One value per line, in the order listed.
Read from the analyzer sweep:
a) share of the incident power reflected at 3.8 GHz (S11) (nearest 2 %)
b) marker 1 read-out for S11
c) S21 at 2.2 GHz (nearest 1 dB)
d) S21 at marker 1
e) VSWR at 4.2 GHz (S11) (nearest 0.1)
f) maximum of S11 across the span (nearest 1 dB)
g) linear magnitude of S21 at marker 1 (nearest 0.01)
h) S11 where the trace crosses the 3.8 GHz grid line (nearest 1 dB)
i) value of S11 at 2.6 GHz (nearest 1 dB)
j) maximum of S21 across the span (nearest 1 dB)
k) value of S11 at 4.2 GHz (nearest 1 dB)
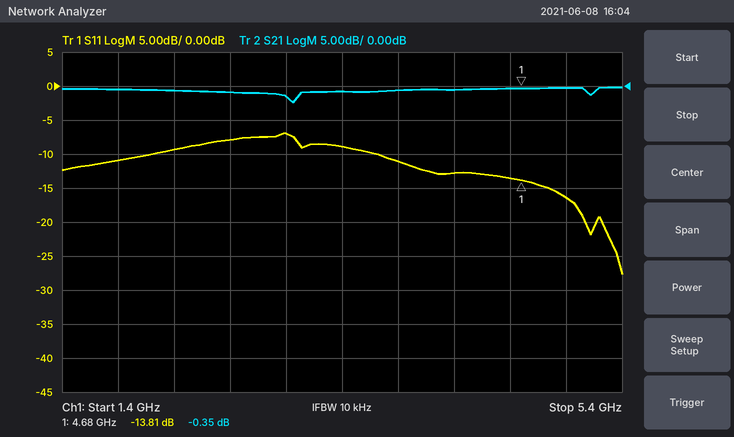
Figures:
8 %
-13.81 dB
-1 dB
-0.35 dB
1.6
-7 dB
0.96
-11 dB
-8 dB
0 dB
-13 dB
